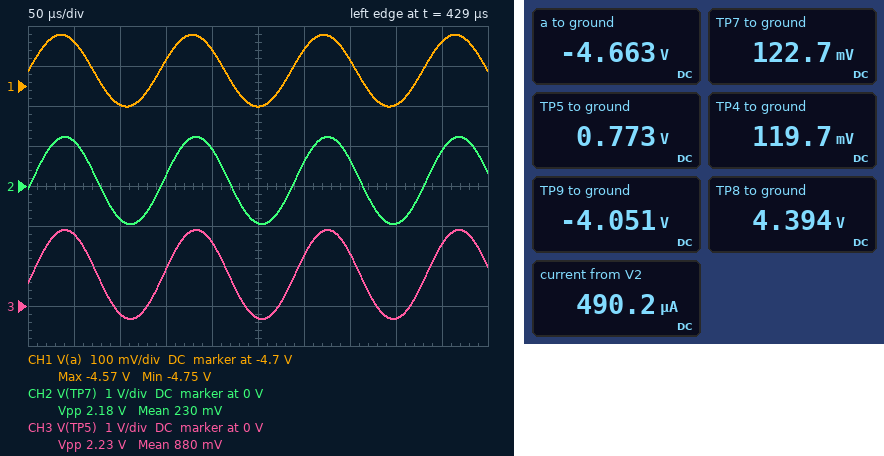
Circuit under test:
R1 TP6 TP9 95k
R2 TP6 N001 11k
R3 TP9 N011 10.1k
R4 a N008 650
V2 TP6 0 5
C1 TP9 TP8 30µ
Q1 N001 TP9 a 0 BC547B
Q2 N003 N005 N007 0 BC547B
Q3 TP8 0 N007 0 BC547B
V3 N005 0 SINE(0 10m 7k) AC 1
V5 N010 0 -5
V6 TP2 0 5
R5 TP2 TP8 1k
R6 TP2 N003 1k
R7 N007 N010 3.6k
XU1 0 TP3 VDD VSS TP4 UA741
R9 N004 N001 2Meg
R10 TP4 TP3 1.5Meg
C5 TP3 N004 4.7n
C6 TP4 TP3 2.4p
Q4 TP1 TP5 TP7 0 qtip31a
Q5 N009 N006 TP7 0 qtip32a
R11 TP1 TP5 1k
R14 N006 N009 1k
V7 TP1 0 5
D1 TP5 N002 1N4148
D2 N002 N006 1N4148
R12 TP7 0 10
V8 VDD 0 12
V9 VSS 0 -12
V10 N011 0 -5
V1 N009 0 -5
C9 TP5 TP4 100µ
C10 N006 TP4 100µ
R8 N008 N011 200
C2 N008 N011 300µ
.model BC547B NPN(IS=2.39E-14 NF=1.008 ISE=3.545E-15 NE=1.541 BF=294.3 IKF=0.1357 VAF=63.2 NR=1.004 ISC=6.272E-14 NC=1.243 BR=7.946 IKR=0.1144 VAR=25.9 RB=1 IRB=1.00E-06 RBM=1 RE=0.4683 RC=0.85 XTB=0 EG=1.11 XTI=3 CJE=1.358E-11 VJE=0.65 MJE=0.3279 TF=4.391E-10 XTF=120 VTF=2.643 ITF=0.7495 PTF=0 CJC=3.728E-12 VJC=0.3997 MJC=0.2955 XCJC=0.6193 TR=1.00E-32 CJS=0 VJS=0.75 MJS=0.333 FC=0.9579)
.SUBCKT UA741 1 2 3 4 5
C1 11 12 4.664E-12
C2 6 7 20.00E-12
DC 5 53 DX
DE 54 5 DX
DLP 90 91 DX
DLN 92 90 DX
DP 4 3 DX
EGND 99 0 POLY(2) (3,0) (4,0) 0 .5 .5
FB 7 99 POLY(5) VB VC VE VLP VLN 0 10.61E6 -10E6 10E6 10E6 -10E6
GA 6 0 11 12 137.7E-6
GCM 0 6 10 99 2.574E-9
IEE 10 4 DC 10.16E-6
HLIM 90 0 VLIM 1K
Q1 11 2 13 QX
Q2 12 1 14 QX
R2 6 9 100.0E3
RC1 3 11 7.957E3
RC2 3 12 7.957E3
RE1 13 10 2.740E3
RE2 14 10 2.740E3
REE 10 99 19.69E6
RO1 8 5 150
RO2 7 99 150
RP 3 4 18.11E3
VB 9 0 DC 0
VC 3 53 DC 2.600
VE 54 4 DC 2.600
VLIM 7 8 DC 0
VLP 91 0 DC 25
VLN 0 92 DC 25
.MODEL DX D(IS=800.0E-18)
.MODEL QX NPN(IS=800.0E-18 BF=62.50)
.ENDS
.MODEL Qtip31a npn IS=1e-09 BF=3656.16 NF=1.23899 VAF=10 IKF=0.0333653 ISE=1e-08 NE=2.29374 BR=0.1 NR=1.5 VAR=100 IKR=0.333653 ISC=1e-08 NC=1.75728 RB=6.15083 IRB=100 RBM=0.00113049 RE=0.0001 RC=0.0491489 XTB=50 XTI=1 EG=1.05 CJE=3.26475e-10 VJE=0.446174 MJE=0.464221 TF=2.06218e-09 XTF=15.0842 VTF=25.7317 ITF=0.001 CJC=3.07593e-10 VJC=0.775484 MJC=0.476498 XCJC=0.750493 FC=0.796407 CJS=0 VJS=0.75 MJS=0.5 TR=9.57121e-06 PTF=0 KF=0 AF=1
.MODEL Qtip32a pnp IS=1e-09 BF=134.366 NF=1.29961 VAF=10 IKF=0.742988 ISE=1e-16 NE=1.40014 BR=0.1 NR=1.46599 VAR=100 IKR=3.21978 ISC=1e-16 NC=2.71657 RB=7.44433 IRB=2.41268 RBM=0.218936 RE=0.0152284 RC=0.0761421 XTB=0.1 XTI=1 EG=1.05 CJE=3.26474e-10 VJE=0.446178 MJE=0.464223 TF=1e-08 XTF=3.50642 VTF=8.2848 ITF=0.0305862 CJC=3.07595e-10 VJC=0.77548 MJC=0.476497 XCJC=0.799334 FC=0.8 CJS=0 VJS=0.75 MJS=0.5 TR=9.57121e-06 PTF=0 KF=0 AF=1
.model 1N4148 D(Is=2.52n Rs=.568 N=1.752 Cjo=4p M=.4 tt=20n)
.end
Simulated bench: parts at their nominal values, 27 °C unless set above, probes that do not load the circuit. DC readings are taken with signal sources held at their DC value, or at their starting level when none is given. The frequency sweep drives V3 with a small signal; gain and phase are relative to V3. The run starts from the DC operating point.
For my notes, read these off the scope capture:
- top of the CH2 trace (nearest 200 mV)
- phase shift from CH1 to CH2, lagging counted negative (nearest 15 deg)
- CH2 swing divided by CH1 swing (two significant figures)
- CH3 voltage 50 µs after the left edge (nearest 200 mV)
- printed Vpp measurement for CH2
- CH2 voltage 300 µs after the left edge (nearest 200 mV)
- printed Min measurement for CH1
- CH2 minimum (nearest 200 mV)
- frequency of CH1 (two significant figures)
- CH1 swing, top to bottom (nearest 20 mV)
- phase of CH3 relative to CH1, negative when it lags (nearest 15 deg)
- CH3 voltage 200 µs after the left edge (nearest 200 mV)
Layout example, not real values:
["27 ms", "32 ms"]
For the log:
["1.2 V", "-15 deg", "12", "1.8 V", "2.18 V", "600 mV", "-4.75 V", "-1.0 V", "7.0 kHz", "180 mV", "-15 deg", "1.6 V"]
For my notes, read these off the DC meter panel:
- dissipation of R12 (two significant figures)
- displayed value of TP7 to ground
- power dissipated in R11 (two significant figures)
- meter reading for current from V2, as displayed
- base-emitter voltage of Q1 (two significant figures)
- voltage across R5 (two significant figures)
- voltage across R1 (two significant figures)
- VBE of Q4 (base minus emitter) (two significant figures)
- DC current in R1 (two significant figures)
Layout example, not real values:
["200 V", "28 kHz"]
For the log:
["1.5 mW", "122.7 mV", "18 mW", "490.2 µA", "610 mV", "610 mV", "9.1 V", "650 mV", "95 µA"]
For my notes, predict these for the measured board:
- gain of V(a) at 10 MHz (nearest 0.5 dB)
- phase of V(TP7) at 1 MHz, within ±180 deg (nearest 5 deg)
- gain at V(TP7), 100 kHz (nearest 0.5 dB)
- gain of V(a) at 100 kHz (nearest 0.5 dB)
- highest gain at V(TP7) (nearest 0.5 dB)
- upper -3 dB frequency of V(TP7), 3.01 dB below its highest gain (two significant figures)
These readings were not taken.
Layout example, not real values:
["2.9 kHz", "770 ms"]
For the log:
["13.0 dB", "90 deg", "32.5 dB", "19.0 dB", "41.0 dB", "40 kHz"]
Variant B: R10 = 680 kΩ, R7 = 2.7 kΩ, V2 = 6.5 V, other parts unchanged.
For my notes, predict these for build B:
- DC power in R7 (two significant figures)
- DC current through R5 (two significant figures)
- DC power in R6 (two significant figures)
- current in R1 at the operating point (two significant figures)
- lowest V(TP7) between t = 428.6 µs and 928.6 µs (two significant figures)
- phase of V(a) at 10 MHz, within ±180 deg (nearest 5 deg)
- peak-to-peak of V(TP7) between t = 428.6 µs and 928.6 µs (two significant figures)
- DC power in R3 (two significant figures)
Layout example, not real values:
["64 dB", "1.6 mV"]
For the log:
["7.1 mW", "810 µA", "650 µW", "110 µA", "-550 mV", "-25 deg", "1.4 V", "120 µW"]
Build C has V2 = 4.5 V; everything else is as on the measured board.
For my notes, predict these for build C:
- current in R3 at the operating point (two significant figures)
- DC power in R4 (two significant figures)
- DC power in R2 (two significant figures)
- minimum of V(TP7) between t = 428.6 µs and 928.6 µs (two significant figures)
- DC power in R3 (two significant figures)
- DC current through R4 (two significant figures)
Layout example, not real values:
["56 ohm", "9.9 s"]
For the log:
["89 µA", "78 µW", "1.3 mW", "-930 mV", "81 µW", "350 µA"]
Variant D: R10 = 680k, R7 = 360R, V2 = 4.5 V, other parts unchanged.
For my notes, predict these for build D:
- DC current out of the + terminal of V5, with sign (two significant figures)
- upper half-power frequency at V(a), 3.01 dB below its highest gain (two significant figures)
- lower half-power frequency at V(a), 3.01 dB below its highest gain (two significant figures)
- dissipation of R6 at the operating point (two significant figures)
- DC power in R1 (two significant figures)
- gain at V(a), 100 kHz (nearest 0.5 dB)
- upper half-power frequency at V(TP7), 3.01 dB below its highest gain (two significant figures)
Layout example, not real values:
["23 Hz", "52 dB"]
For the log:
["-12 mA", "200 MHz", "620 mHz", "32 mW", "780 µW", "2.5 dB", "92 kHz"]
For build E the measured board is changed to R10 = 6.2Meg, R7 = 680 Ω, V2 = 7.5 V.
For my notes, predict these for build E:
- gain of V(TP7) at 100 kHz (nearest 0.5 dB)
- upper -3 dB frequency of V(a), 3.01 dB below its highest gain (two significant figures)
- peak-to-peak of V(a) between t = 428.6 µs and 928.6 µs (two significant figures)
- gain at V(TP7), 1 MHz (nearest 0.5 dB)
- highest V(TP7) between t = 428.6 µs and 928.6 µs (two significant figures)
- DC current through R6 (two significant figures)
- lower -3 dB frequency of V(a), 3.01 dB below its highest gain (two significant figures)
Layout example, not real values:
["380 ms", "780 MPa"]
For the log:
["47.0 dB", "3.8 MHz", "740 mV", "17.5 dB", "4.8 V", "3.2 mA", "530 mHz"]
